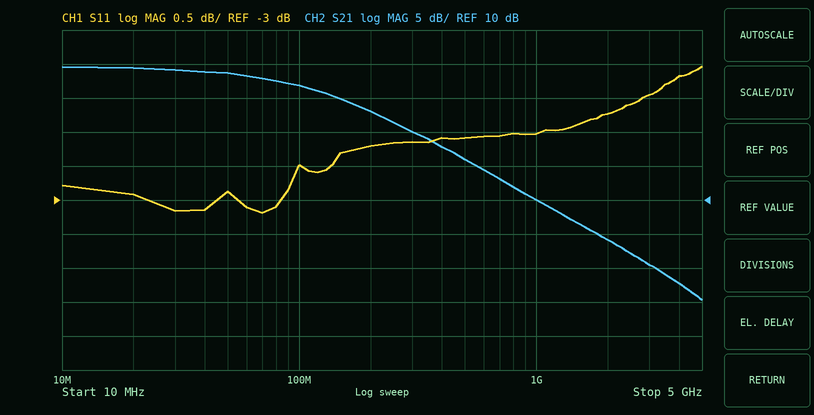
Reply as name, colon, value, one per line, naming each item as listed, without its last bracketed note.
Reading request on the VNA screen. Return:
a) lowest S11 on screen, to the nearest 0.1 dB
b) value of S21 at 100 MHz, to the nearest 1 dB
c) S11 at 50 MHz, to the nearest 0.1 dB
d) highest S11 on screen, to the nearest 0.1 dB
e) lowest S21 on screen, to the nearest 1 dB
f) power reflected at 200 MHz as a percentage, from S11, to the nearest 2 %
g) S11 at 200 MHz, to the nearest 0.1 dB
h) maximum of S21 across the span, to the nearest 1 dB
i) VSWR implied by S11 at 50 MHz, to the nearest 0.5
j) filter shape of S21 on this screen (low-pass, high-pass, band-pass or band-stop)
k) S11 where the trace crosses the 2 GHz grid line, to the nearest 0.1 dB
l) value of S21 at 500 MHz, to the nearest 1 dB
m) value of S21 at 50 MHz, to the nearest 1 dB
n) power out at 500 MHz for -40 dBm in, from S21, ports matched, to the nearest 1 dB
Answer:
lowest S11 on screen, to the nearest 0.1 dB: -3.2 dB
value of S21 at 100 MHz, to the nearest 1 dB: 27 dB
S11 at 50 MHz, to the nearest 0.1 dB: -2.9 dB
highest S11 on screen, to the nearest 0.1 dB: -1.0 dB
lowest S21 on screen, to the nearest 1 dB: -5 dB
power reflected at 200 MHz as a percentage, from S11, to the nearest 2 %: 60 %
S11 at 200 MHz, to the nearest 0.1 dB: -2.2 dB
maximum of S21 across the span, to the nearest 1 dB: 30 dB
VSWR implied by S11 at 50 MHz, to the nearest 0.5: 6.0
filter shape of S21 on this screen: low-pass
S11 where the trace crosses the 2 GHz grid line, to the nearest 0.1 dB: -1.7 dB
value of S21 at 500 MHz, to the nearest 1 dB: 16 dB
value of S21 at 50 MHz, to the nearest 1 dB: 29 dB
power out at 500 MHz for -40 dBm in, from S21, ports matched, to the nearest 1 dB: -24 dBm
